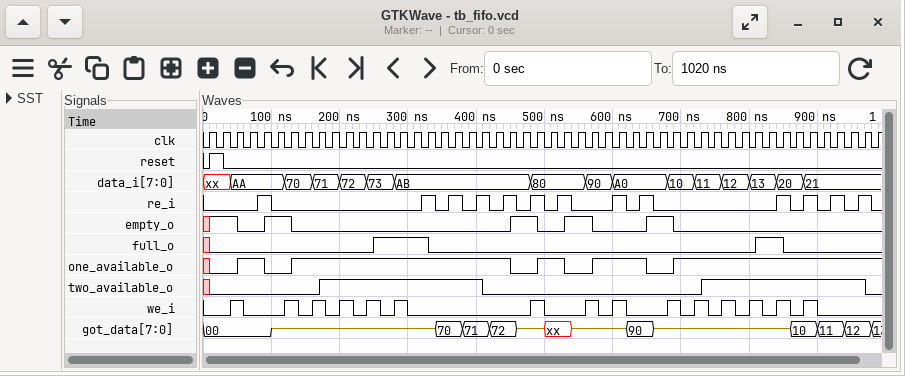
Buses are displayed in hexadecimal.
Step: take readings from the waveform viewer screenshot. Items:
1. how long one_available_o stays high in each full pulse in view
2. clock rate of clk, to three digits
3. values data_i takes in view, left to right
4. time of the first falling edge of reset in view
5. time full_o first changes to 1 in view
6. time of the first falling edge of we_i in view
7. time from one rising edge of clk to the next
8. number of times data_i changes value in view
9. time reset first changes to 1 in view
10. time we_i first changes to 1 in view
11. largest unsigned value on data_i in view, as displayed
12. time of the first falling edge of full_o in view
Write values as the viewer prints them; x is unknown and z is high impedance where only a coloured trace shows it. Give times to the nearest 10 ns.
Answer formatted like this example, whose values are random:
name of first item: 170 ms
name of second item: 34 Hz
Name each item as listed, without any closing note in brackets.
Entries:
how long one_available_o stays high in each full pulse in view: 40 ns, 320 ns, 40 ns, 80 ns
clock rate of clk, to three digits: 50.0 MHz
values data_i takes in view, left to right: xx, AA, 70, 71, 72, 73, AB, 80, 90, A0, 10, 11, 12, 13, 20, 21
time of the first falling edge of reset in view: 30 ns
time full_o first changes to 1 in view: 250 ns
time of the first falling edge of we_i in view: 60 ns
time from one rising edge of clk to the next: 20 ns
number of times data_i changes value in view: 15
time reset first changes to 1 in view: 10 ns
time we_i first changes to 1 in view: 40 ns
largest unsigned value on data_i in view, as displayed: AB
time of the first falling edge of full_o in view: 330 ns
